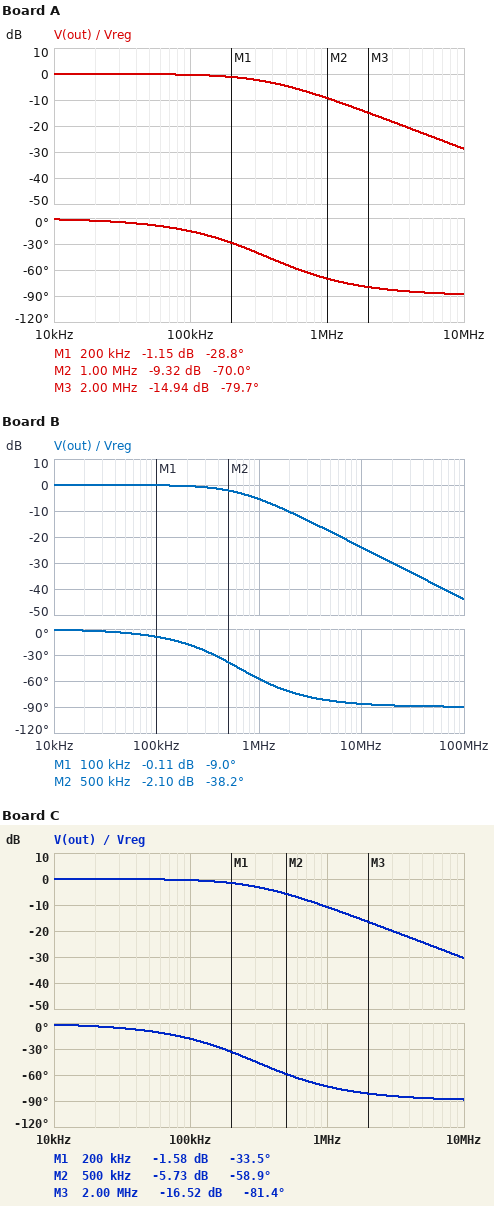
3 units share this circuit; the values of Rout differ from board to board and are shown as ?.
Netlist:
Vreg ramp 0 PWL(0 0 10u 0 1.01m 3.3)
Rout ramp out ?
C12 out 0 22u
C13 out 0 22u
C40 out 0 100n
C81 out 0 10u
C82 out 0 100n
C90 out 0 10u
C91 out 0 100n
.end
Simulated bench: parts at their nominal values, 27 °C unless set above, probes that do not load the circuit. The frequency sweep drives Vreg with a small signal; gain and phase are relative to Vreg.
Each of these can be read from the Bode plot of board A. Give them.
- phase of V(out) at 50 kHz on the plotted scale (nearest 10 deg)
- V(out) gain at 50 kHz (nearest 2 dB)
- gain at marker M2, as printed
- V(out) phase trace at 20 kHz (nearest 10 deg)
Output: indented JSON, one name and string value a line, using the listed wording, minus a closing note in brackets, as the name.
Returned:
{
  "phase of V(out) at 50 kHz on the plotted scale": "-10 deg",
  "V(out) gain at 50 kHz": "0 dB",
  "gain at marker M2, as printed": "-9.32 dB",
  "V(out) phase trace at 20 kHz": "0 deg"
}
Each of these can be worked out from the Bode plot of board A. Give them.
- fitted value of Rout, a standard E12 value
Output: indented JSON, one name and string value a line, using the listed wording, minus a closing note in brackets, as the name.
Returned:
{
  "fitted value of Rout, a standard E12 value": "6.8 mΩ"
}
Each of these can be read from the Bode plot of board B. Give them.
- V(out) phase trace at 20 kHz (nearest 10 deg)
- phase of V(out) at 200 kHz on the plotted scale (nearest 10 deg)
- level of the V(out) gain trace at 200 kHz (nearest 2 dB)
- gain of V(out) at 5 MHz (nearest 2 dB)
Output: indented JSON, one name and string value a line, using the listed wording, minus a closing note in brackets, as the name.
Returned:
{
  "V(out) phase trace at 20 kHz": "0 deg",
  "phase of V(out) at 200 kHz on the plotted scale": "-20 deg",
  "level of the V(out) gain trace at 200 kHz": "0 dB",
  "gain of V(out) at 5 MHz": "-18 dB"
}
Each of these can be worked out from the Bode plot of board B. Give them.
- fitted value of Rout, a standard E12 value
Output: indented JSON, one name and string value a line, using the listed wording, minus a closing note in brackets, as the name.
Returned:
{
  "fitted value of Rout, a standard E12 value": "3.9 mΩ"
}
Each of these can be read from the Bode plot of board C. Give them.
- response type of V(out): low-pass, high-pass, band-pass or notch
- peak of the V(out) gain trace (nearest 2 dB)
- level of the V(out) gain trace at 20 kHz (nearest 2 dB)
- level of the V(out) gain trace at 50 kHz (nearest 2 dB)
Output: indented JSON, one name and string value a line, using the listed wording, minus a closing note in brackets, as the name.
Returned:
{
  "response type of V(out): low-pass, high-pass, band-pass or notch": "low-pass",
  "peak of the V(out) gain trace": "0 dB",
  "level of the V(out) gain trace at 20 kHz": "0 dB",
  "level of the V(out) gain trace at 50 kHz": "0 dB"
}
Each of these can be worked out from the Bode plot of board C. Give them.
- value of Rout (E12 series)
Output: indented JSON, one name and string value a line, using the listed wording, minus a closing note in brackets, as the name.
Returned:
{
  "value of Rout": "8.2 mΩ"
}
